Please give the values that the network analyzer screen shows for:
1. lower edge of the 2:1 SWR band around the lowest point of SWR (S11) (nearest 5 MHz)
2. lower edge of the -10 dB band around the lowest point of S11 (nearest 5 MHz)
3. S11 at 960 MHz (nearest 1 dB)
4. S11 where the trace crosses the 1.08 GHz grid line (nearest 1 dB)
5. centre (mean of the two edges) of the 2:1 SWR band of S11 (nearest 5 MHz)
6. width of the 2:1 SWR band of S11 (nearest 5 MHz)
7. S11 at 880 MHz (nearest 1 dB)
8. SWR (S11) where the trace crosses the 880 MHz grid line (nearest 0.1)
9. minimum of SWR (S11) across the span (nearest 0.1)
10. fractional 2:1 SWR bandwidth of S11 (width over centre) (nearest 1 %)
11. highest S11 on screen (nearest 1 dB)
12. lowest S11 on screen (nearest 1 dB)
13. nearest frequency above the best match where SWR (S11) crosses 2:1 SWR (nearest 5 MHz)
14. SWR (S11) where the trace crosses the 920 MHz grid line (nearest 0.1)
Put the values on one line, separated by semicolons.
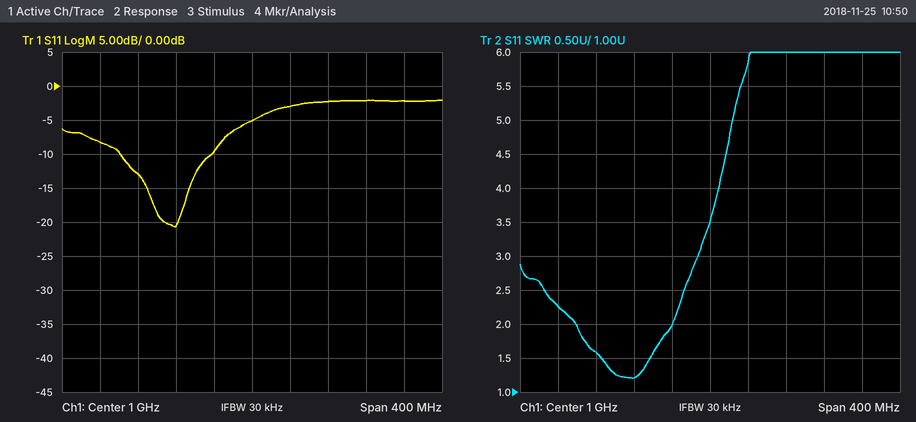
860 MHz; 860 MHz; -10 dB; -2 dB; 910 MHz; 100 MHz; -13 dB; 1.6; 1.2; 11 %; -2 dB; -21 dB; 960 MHz; 1.2
